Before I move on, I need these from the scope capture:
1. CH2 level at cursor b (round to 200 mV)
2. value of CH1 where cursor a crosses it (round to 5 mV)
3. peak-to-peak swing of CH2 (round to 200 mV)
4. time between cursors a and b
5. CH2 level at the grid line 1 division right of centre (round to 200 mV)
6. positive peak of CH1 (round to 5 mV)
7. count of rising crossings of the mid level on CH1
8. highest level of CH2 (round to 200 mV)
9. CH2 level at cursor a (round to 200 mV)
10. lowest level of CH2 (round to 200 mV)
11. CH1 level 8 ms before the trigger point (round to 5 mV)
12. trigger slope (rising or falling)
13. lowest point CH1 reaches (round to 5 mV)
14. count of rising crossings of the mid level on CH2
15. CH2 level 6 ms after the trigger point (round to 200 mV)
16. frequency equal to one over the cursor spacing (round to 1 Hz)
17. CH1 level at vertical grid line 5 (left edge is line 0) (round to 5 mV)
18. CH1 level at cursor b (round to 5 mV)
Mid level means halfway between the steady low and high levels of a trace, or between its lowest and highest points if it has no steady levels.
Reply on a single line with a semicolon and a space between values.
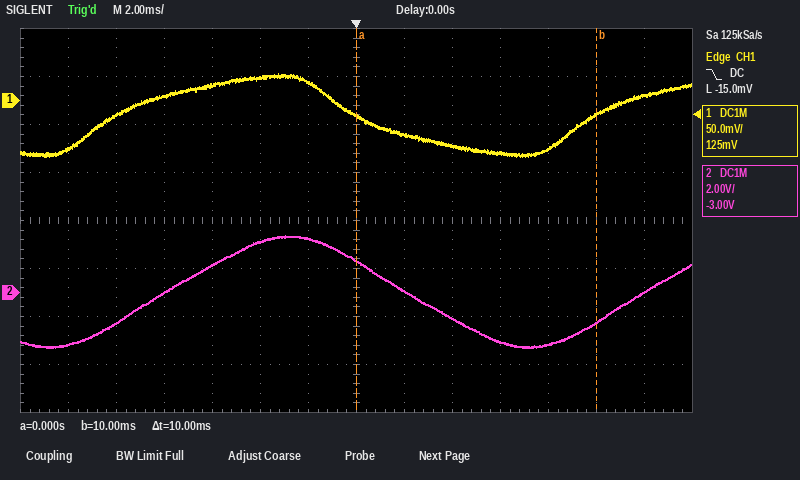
-1.2 V; -15 mV; 4.6 V; 10 ms; 0.0 V; 30 mV; 2; 2.4 V; 1.4 V; -2.2 V; 5 mV; falling; -60 mV; 2; -2.0 V; 100 Hz; 25 mV; -15 mV
